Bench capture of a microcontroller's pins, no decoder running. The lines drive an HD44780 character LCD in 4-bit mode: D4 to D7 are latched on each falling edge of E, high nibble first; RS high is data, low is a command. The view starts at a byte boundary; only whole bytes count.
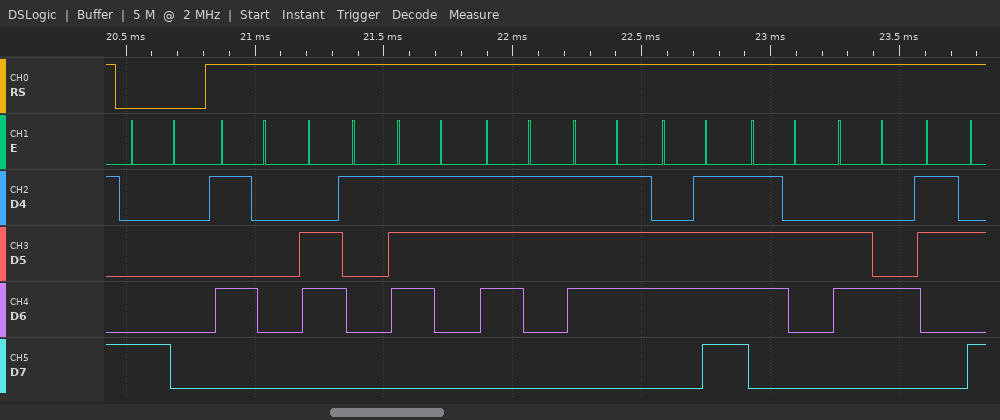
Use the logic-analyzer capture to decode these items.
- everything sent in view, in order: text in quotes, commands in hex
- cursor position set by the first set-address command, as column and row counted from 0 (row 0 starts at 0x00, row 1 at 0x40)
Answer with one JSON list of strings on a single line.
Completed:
["0x80 \"Password:\"", "column 0, row 0"]
